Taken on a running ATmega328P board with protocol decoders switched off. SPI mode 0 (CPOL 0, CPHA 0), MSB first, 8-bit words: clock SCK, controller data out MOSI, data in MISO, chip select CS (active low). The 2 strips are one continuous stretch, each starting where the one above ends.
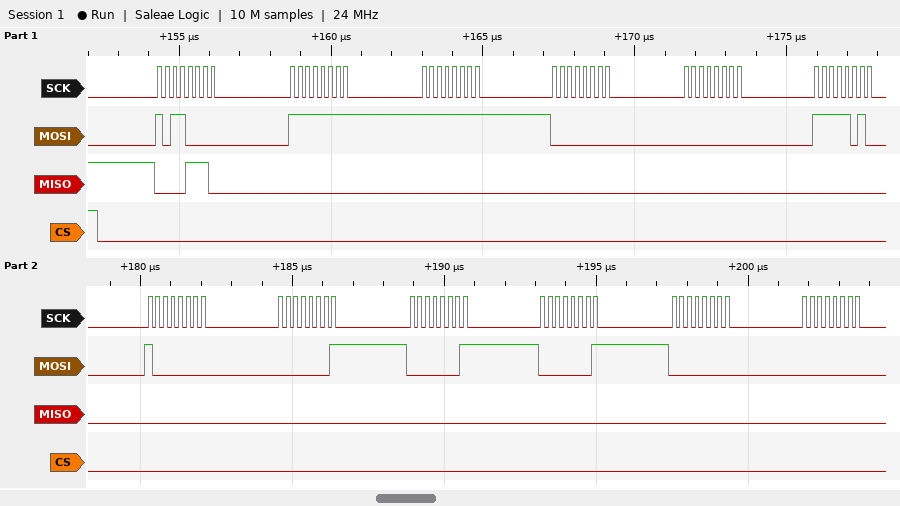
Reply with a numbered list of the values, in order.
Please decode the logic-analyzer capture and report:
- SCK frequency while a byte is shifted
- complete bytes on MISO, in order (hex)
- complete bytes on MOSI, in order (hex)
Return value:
1. 4 MHz
2. 0E 00 00 00 00 00 00 00 00 00 00 00
3. B0 FF FF 00 00 FA 80 01 01 01 00 00
